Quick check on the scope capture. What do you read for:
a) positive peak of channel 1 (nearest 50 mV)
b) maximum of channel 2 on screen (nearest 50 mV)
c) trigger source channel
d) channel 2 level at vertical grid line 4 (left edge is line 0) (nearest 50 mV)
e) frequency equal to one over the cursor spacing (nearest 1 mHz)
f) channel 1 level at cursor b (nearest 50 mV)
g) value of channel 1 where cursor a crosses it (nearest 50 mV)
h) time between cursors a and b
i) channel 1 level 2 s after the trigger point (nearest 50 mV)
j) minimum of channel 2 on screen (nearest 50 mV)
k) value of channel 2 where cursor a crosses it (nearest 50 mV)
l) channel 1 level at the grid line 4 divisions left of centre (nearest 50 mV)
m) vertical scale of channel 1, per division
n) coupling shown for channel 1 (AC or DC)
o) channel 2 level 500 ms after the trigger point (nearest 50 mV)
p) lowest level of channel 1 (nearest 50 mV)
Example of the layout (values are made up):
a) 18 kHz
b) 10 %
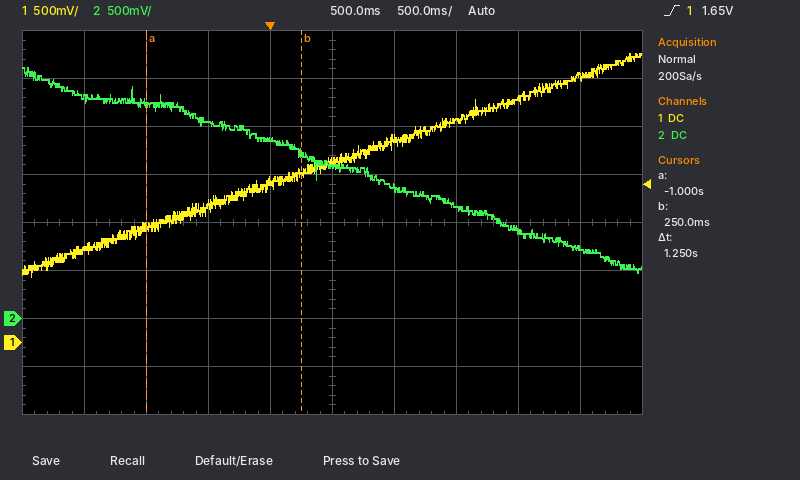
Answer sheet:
a) 3.00 V
b) 2.60 V
c) channel 1
d) 1.85 V
e) 800 mHz
f) 1.75 V
g) 1.20 V
h) 1.25 s
i) 2.55 V
j) 500 mV
k) 2.25 V
l) 950 mV
m) 500 mV
n) DC
o) 1.60 V
p) 700 mV
